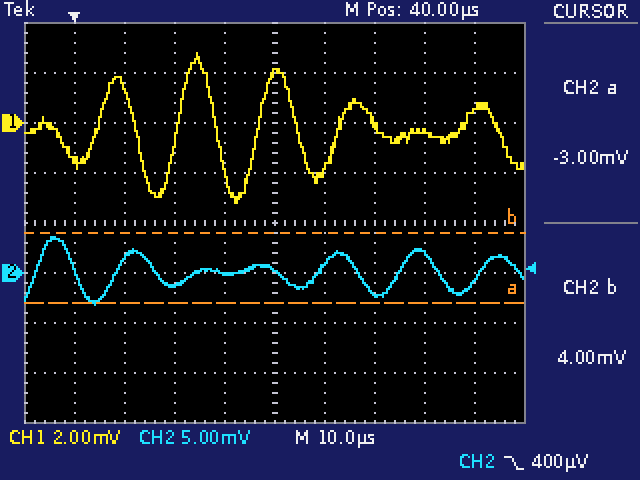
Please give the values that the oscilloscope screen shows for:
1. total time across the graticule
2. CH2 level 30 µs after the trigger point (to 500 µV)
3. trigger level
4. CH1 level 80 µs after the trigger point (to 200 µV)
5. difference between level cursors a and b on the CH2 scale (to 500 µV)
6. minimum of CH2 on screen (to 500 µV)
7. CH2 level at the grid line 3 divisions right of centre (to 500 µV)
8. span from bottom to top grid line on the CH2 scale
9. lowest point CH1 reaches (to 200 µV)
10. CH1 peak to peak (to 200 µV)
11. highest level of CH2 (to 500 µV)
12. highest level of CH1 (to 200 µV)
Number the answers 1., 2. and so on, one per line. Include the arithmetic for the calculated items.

1. 100 µs
2. 0.0 mV
3. 400 µV
4. 600 µV
5. 7.0 mV
6. -3.0 mV
7. 2.0 mV
8. 40 mV
9. -3.2 mV
10. 2.8 mV − (-3.2 mV) = 6.0 mV
11. 3.5 mV
12. 2.8 mV
